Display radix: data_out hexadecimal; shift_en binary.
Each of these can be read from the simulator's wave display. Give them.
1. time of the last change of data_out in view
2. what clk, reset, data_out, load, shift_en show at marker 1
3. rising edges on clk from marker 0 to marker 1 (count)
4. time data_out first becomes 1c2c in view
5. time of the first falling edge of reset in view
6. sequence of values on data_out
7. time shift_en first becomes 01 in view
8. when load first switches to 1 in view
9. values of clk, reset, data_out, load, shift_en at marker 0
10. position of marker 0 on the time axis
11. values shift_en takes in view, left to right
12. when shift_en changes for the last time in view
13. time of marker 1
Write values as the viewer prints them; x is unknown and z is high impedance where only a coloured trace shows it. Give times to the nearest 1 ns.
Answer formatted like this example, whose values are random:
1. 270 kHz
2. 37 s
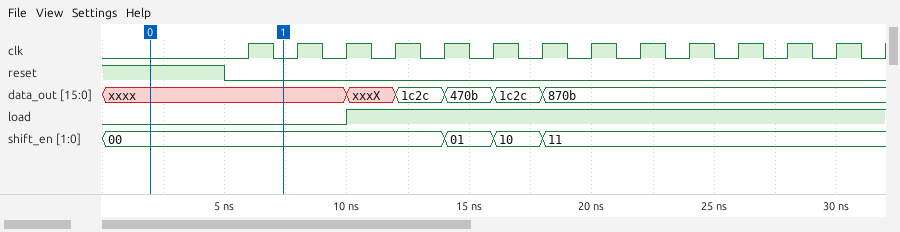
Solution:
1. 18 ns
2. clk=0, reset=0, data_out=xxxx, load=0, shift_en=00
3. 1
4. 12 ns
5. 5 ns
6. xxxx, xxxX, 1c2c, 470b, 1c2c, 870b
7. 14 ns
8. 10 ns
9. clk=0, reset=1, data_out=xxxx, load=0, shift_en=00
10. 2 ns
11. 00, 01, 10, 11
12. 18 ns
13. 7 ns
